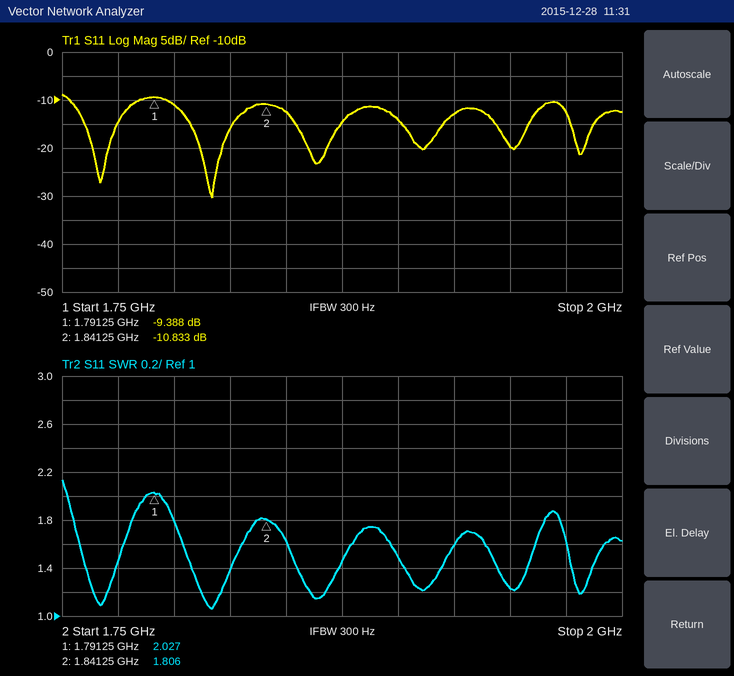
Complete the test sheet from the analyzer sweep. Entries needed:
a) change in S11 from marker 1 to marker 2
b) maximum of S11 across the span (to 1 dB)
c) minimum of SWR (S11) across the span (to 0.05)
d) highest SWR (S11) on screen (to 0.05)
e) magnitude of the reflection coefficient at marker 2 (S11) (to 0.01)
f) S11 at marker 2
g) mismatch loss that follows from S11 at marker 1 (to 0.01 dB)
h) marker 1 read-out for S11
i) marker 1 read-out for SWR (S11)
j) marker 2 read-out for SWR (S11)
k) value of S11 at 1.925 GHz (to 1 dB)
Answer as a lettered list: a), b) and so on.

a) -1.445 dB
b) -9 dB
c) 1.05
d) 2.15
e) 0.29
f) -10.833 dB
g) 0.53 dB
h) -9.388 dB
i) 2.027
j) 1.806
k) -13 dB
